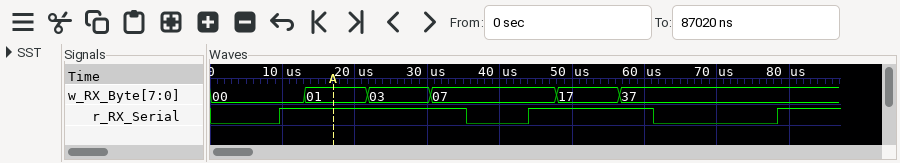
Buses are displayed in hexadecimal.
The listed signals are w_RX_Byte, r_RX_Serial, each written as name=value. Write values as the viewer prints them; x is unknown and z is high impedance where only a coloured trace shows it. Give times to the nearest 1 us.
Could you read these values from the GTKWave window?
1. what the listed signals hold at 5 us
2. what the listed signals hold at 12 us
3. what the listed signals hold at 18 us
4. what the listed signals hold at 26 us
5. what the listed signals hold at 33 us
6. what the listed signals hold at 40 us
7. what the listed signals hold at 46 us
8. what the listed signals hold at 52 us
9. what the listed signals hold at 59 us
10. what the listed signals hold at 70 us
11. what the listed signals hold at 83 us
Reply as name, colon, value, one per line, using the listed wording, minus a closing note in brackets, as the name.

what the listed signals hold at 5 us: w_RX_Byte=00, r_RX_Serial=0
what the listed signals hold at 12 us: w_RX_Byte=00, r_RX_Serial=1
what the listed signals hold at 18 us: w_RX_Byte=01, r_RX_Serial=1
what the listed signals hold at 26 us: w_RX_Byte=03, r_RX_Serial=1
what the listed signals hold at 33 us: w_RX_Byte=07, r_RX_Serial=1
what the listed signals hold at 40 us: w_RX_Byte=07, r_RX_Serial=0
what the listed signals hold at 46 us: w_RX_Byte=07, r_RX_Serial=1
what the listed signals hold at 52 us: w_RX_Byte=17, r_RX_Serial=1
what the listed signals hold at 59 us: w_RX_Byte=37, r_RX_Serial=1
what the listed signals hold at 70 us: w_RX_Byte=37, r_RX_Serial=0
what the listed signals hold at 83 us: w_RX_Byte=37, r_RX_Serial=1
